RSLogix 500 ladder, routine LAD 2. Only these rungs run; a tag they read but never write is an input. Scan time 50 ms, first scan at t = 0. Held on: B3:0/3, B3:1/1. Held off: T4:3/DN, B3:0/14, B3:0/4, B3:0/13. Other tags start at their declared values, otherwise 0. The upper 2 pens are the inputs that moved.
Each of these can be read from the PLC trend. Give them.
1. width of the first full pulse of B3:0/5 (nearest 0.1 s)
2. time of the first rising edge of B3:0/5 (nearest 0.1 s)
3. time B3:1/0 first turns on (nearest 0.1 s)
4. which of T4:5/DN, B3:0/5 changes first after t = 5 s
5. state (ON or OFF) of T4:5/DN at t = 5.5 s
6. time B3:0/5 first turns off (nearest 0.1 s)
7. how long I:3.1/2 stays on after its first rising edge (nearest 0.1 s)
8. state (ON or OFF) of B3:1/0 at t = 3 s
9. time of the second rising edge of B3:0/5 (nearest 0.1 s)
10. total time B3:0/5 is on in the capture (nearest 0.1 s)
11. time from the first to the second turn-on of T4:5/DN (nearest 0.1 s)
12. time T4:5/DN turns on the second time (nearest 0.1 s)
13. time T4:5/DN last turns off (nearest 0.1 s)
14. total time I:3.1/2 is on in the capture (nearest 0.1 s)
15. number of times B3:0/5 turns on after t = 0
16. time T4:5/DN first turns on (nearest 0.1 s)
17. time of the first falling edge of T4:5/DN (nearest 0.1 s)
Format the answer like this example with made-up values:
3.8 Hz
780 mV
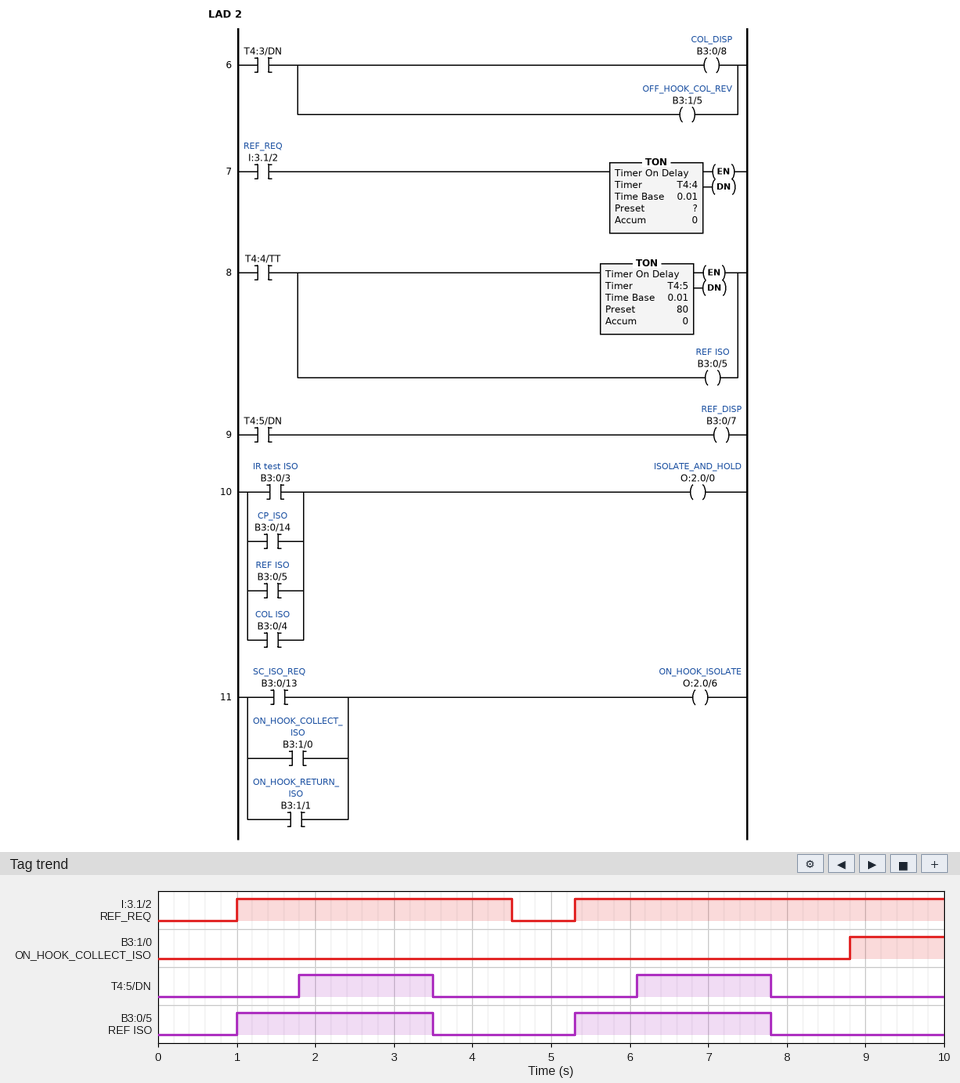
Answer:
2.5 s
1.0 s
8.8 s
B3:0/5
OFF
3.5 s
3.5 s
OFF
5.3 s
5.0 s
4.3 s
6.1 s
7.8 s
8.2 s
2
1.8 s
3.5 s
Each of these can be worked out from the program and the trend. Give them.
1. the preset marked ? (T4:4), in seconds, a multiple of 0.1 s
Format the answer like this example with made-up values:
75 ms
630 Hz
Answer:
2.5 s
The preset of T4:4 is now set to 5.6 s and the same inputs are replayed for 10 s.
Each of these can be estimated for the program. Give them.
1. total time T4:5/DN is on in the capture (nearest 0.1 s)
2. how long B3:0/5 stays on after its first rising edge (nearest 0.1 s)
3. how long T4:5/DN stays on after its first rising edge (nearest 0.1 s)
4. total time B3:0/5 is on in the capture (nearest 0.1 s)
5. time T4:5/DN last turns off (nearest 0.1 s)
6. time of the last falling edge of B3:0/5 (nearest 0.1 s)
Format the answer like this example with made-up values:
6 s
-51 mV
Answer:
6.6 s
3.5 s
2.7 s
8.2 s
4.5 s
4.5 s
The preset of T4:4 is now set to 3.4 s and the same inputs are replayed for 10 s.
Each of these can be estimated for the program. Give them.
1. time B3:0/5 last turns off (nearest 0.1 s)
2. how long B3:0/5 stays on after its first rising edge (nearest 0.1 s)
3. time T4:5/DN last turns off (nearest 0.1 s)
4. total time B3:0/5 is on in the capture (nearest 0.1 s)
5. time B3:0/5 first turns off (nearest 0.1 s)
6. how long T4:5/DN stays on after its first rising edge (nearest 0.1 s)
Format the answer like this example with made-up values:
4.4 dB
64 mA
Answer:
8.7 s
3.4 s
8.7 s
6.8 s
4.4 s
2.6 s
